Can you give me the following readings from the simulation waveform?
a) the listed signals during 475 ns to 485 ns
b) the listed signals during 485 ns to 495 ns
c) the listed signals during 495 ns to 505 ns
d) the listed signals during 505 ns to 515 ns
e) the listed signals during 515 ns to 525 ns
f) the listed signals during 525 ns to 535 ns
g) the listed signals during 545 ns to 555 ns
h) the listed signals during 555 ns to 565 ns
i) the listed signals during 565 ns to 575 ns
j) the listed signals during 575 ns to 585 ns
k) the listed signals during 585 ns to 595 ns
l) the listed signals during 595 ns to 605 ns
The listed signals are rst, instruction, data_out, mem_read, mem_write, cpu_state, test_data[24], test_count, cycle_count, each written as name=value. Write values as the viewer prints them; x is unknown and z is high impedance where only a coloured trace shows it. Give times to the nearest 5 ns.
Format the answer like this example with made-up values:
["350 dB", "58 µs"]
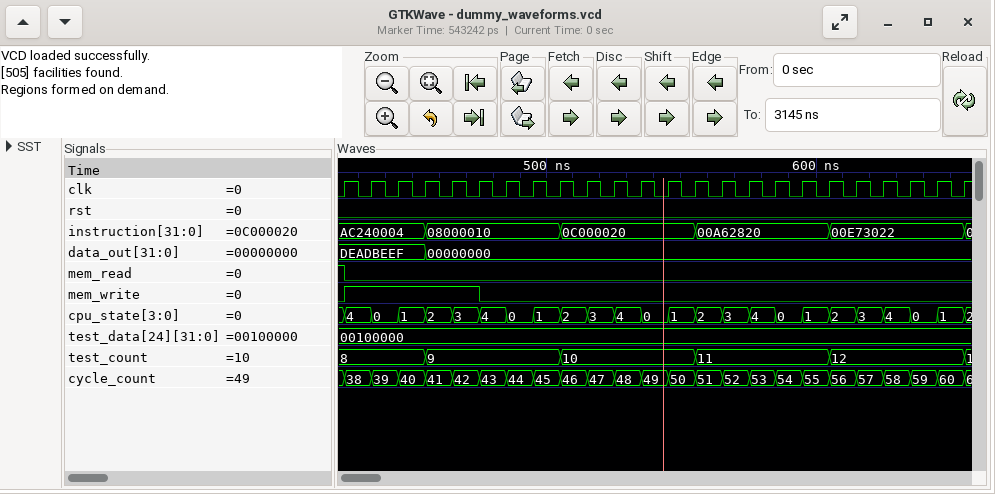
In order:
["rst=0, instruction=08000010, data_out=00000000, mem_read=0, mem_write=0, cpu_state=4, test_data[24]=00100000, test_count=9, cycle_count=43", "rst=0, instruction=08000010, data_out=00000000, mem_read=0, mem_write=0, cpu_state=0, test_data[24]=00100000, test_count=9, cycle_count=44", "rst=0, instruction=08000010, data_out=00000000, mem_read=0, mem_write=0, cpu_state=1, test_data[24]=00100000, test_count=9, cycle_count=45", "rst=0, instruction=0C000020, data_out=00000000, mem_read=0, mem_write=0, cpu_state=2, test_data[24]=00100000, test_count=10, cycle_count=46", "rst=0, instruction=0C000020, data_out=00000000, mem_read=0, mem_write=0, cpu_state=3, test_data[24]=00100000, test_count=10, cycle_count=47", "rst=0, instruction=0C000020, data_out=00000000, mem_read=0, mem_write=0, cpu_state=4, test_data[24]=00100000, test_count=10, cycle_count=48", "rst=0, instruction=0C000020, data_out=00000000, mem_read=0, mem_write=0, cpu_state=1, test_data[24]=00100000, test_count=10, cycle_count=50", "rst=0, instruction=00A62820, data_out=00000000, mem_read=0, mem_write=0, cpu_state=2, test_data[24]=00100000, test_count=11, cycle_count=51", "rst=0, instruction=00A62820, data_out=00000000, mem_read=0, mem_write=0, cpu_state=3, test_data[24]=00100000, test_count=11, cycle_count=52", "rst=0, instruction=00A62820, data_out=00000000, mem_read=0, mem_write=0, cpu_state=4, test_data[24]=00100000, test_count=11, cycle_count=53", "rst=0, instruction=00A62820, data_out=00000000, mem_read=0, mem_write=0, cpu_state=0, test_data[24]=00100000, test_count=11, cycle_count=54", "rst=0, instruction=00A62820, data_out=00000000, mem_read=0, mem_write=0, cpu_state=1, test_data[24]=00100000, test_count=11, cycle_count=55"]
